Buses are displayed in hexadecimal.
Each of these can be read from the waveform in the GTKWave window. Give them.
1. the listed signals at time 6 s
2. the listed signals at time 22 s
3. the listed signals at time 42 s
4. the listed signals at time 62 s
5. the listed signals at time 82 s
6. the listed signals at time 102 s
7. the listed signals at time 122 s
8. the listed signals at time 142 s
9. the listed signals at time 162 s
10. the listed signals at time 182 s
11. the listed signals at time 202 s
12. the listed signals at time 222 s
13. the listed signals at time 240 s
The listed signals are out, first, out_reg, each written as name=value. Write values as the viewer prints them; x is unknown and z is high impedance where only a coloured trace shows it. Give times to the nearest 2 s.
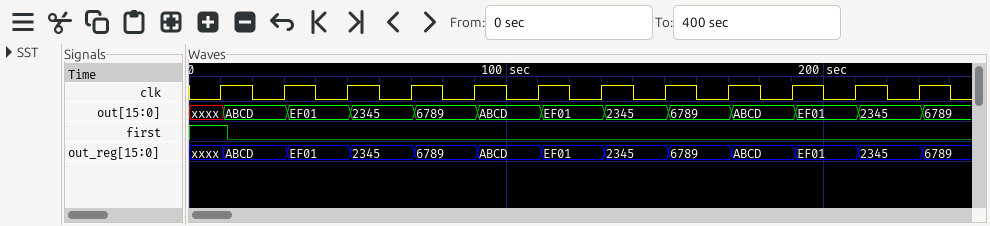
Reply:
out=xxxx, first=1, out_reg=xxxx
out=ABCD, first=0, out_reg=ABCD
out=EF01, first=0, out_reg=EF01
out=2345, first=0, out_reg=2345
out=6789, first=0, out_reg=6789
out=ABCD, first=0, out_reg=ABCD
out=EF01, first=0, out_reg=EF01
out=2345, first=0, out_reg=2345
out=6789, first=0, out_reg=6789
out=ABCD, first=0, out_reg=ABCD
out=EF01, first=0, out_reg=EF01
out=2345, first=0, out_reg=2345
out=6789, first=0, out_reg=6789
